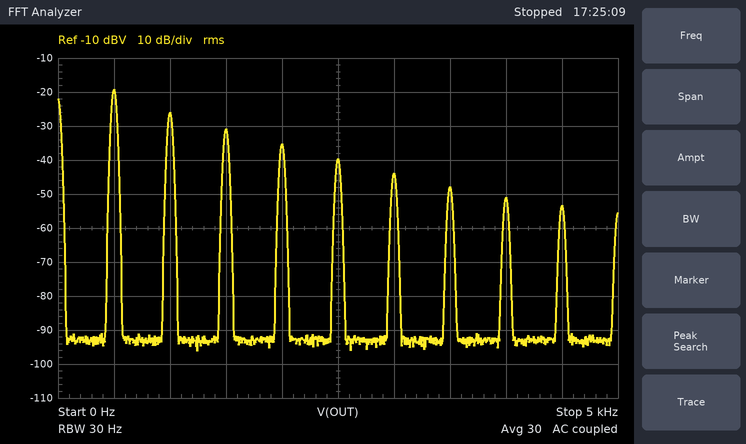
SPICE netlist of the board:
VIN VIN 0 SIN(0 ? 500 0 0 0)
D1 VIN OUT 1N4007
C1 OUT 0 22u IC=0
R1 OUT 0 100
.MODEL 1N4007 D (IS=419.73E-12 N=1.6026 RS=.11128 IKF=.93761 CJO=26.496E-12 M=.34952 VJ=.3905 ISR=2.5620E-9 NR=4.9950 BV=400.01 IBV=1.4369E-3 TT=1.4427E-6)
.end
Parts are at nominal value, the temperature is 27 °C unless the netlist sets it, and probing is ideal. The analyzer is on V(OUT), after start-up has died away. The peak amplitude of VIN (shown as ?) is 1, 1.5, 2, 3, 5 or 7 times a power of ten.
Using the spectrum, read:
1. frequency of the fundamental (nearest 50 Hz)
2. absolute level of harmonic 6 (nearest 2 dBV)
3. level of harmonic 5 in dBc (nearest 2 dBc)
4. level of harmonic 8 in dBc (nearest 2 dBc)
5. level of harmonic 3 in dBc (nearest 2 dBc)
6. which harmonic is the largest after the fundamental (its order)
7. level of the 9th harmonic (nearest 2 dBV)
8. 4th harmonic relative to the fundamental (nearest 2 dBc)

500 Hz
-44 dBV
-20 dBc
-32 dBc
-12 dBc
2
-54 dBV
-16 dBc
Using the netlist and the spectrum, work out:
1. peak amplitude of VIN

1.5 V
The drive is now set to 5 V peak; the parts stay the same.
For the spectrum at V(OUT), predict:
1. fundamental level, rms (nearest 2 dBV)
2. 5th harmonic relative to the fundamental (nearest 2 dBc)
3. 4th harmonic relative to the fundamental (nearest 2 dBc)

-4 dBV
-22 dBc
-18 dBc
